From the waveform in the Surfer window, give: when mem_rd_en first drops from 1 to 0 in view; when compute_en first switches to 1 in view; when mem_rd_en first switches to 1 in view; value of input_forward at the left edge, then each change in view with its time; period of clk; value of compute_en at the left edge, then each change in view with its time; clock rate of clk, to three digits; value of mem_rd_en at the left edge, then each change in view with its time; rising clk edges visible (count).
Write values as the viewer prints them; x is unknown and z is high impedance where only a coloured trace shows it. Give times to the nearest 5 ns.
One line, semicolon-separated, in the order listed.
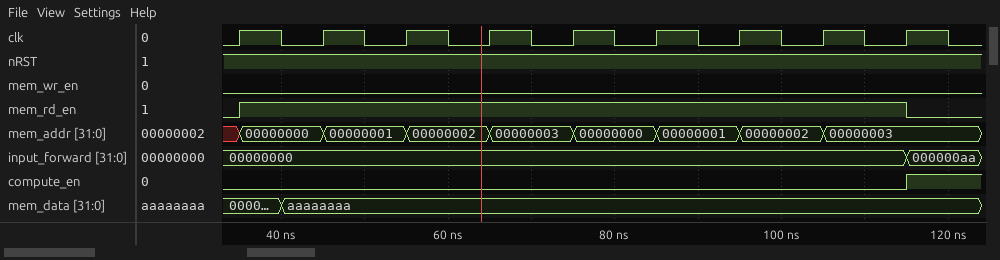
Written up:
115 ns; 115 ns; 35 ns; 00000000, 000000aa at 115 ns; 10 ns; 0, 1 at 115 ns; 100 MHz; 0, 1 at 35 ns, 0 at 115 ns; 9
